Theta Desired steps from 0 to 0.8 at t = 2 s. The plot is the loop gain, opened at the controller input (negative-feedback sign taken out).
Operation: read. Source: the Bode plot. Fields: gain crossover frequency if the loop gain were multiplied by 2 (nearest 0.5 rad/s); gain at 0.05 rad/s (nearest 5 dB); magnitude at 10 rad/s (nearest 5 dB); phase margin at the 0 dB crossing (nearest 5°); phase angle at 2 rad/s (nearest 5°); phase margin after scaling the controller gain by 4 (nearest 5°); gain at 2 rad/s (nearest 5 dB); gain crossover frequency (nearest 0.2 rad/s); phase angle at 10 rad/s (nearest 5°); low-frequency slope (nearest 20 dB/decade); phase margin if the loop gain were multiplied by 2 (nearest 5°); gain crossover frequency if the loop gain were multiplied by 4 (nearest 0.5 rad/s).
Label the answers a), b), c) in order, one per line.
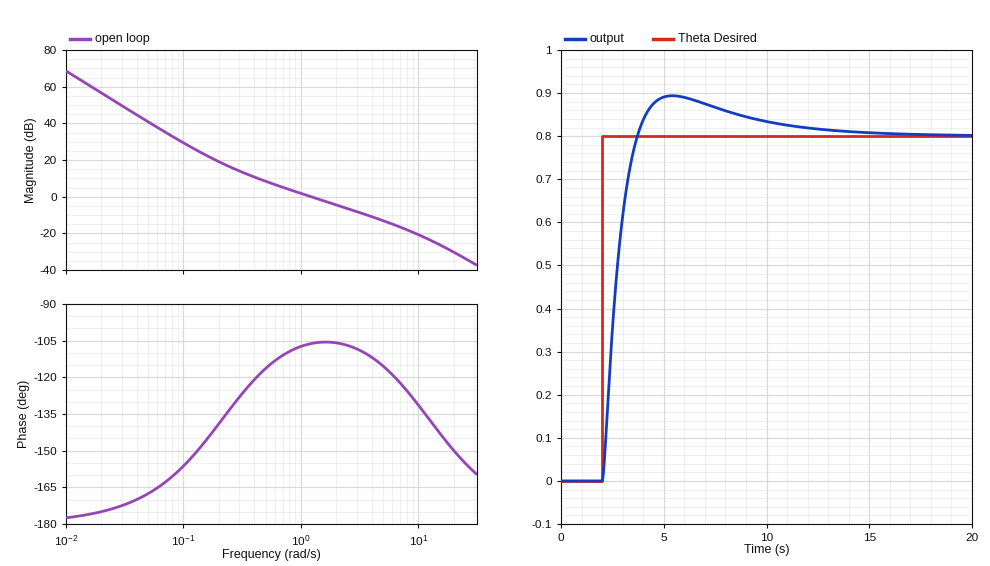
a) 2.5 rad/s
b) 40 dB
c) -20 dB
d) 75°
e) -105°
f) 65°
g) -5 dB
h) 1.2 rad/s
i) -130°
j) -40 dB/decade
k) 75°
l) 4.5 rad/s
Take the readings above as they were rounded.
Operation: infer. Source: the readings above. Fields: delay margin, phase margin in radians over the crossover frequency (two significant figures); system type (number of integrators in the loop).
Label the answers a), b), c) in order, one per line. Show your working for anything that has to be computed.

a) 75 × π / 180 / 1.2 = 1.1 s
b) 2
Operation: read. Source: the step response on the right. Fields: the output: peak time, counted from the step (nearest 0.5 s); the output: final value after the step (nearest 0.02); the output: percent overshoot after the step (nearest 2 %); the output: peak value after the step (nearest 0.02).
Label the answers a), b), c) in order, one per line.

a) 3.5 s
b) 0.80
c) 12 %
d) 0.90
